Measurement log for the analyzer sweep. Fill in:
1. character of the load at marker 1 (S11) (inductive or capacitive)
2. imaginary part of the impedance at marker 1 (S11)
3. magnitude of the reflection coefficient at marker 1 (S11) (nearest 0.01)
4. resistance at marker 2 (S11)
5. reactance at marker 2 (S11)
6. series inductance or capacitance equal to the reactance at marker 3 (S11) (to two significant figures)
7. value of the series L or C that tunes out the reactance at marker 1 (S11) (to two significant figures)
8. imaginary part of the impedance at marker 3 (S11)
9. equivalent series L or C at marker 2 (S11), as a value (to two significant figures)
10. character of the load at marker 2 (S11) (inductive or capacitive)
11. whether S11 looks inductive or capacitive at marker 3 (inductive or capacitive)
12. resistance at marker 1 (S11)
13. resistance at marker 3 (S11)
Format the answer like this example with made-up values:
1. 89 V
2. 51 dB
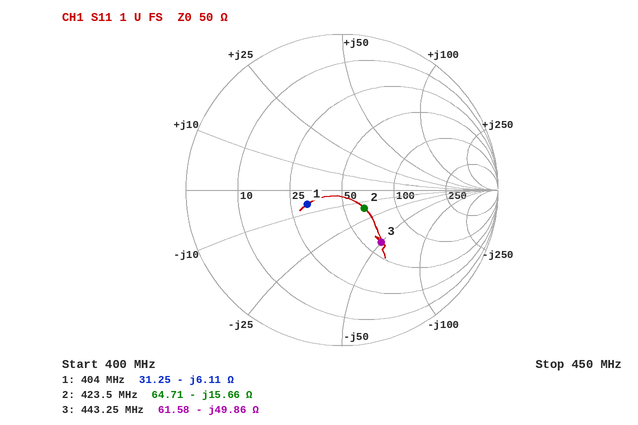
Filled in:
1. capacitive
2. -6.11 Ω
3. 0.24
4. 64.71 Ω
5. -15.66 Ω
6. 7.2 pF
7. 2.4 nH
8. -49.86 Ω
9. 24 pF
10. capacitive
11. capacitive
12. 31.25 Ω
13. 61.58 Ω
